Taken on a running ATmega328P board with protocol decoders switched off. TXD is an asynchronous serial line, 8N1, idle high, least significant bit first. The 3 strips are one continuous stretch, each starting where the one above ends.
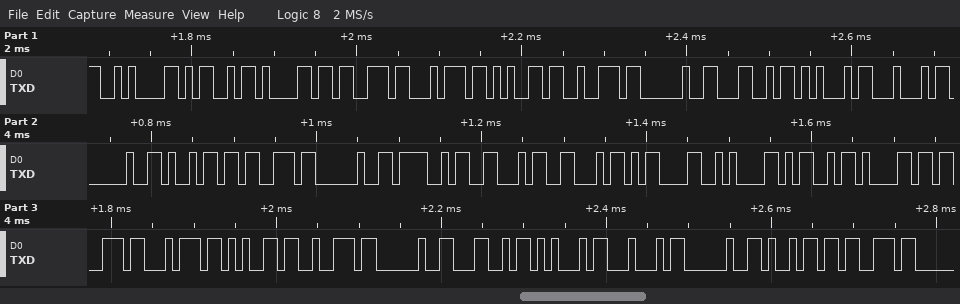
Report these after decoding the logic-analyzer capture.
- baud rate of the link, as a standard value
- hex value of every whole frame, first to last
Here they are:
115200 baud
0A 4D 61 73 74 65 72 20 4C 45 44 20 69 73 20 4F 46 46 0D 0A 4D 61 73 74 65 72 20 4C 45 44 20 69 73
